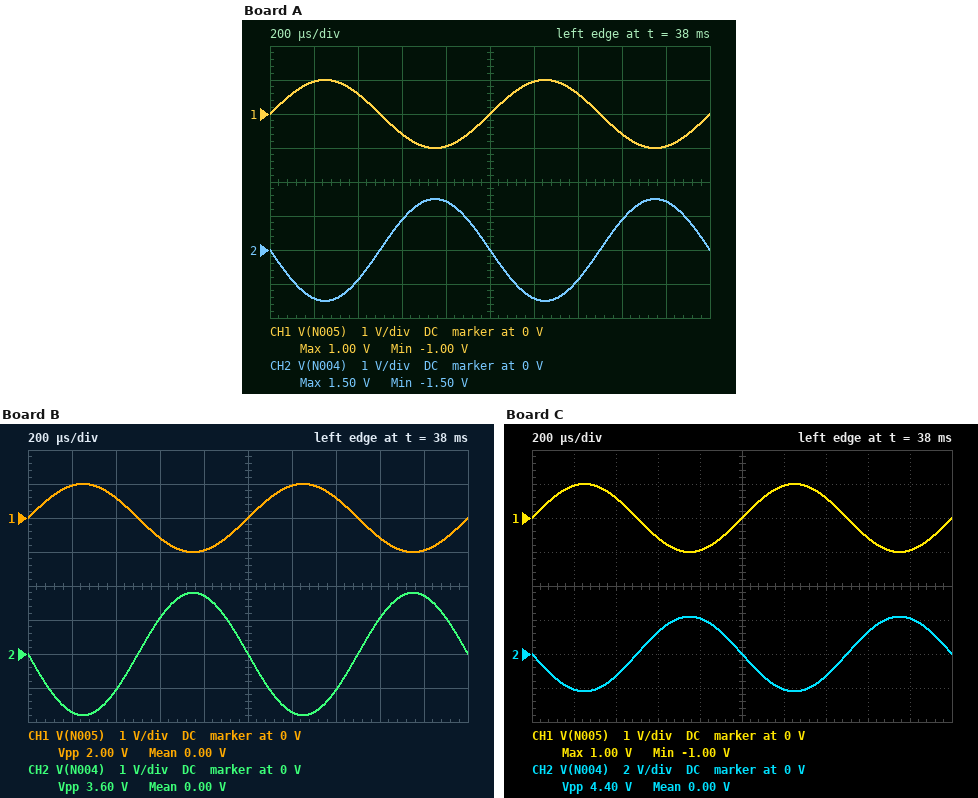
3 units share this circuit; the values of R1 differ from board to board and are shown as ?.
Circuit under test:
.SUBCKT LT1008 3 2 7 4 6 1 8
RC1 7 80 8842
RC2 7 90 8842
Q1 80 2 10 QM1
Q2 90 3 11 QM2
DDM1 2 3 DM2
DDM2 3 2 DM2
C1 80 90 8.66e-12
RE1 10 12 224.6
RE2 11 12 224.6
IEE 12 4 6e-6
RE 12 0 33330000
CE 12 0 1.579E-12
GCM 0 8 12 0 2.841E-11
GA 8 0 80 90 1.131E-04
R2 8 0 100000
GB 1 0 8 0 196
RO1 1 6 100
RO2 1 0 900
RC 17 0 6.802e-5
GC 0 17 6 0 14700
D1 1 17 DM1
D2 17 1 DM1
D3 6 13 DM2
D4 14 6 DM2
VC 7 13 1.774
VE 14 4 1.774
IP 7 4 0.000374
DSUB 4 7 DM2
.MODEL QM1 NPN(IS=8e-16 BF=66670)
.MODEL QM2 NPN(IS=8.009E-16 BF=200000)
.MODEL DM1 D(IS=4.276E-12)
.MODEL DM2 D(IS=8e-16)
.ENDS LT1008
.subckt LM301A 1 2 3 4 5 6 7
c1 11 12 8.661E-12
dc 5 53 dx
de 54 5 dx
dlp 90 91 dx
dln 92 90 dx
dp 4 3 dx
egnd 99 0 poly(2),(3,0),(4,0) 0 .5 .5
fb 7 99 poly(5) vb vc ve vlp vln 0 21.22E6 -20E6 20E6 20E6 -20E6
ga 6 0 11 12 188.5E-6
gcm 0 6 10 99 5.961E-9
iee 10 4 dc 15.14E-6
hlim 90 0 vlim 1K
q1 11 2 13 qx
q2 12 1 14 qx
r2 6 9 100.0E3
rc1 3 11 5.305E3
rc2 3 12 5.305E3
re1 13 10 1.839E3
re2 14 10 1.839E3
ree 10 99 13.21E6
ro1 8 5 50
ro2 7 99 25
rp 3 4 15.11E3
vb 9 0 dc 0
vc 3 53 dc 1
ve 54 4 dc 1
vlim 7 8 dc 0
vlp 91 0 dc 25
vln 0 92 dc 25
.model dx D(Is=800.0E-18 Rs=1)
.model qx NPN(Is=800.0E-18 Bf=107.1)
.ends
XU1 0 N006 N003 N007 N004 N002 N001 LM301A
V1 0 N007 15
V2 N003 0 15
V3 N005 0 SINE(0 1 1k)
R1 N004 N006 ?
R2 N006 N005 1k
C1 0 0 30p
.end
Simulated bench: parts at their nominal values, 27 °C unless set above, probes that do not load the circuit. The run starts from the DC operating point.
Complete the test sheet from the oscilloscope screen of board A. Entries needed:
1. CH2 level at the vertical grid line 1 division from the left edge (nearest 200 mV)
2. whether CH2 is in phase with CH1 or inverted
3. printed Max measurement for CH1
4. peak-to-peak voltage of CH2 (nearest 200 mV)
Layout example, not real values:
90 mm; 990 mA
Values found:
-1.4 V; inverted; 1.00 V; 3.0 V
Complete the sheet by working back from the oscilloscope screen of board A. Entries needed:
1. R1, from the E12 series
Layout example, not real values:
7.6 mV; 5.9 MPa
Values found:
1.5 kΩ
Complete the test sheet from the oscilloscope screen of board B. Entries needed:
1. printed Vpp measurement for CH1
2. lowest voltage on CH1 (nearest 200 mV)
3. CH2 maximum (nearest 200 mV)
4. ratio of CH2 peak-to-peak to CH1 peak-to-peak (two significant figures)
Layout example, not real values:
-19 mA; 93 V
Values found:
2.00 V; -1.0 V; 1.8 V; 1.8
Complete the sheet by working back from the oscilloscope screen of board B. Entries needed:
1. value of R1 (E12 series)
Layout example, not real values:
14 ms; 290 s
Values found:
1.8 kΩ
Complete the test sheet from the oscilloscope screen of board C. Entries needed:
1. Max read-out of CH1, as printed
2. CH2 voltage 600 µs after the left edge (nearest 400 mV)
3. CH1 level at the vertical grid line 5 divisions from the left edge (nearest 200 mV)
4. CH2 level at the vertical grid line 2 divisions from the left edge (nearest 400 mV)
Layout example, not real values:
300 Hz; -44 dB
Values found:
1.00 V; 1.2 V; 0 V; -1.2 V
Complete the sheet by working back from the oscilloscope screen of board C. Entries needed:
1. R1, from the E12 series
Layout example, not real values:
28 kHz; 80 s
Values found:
2.2 kΩ
